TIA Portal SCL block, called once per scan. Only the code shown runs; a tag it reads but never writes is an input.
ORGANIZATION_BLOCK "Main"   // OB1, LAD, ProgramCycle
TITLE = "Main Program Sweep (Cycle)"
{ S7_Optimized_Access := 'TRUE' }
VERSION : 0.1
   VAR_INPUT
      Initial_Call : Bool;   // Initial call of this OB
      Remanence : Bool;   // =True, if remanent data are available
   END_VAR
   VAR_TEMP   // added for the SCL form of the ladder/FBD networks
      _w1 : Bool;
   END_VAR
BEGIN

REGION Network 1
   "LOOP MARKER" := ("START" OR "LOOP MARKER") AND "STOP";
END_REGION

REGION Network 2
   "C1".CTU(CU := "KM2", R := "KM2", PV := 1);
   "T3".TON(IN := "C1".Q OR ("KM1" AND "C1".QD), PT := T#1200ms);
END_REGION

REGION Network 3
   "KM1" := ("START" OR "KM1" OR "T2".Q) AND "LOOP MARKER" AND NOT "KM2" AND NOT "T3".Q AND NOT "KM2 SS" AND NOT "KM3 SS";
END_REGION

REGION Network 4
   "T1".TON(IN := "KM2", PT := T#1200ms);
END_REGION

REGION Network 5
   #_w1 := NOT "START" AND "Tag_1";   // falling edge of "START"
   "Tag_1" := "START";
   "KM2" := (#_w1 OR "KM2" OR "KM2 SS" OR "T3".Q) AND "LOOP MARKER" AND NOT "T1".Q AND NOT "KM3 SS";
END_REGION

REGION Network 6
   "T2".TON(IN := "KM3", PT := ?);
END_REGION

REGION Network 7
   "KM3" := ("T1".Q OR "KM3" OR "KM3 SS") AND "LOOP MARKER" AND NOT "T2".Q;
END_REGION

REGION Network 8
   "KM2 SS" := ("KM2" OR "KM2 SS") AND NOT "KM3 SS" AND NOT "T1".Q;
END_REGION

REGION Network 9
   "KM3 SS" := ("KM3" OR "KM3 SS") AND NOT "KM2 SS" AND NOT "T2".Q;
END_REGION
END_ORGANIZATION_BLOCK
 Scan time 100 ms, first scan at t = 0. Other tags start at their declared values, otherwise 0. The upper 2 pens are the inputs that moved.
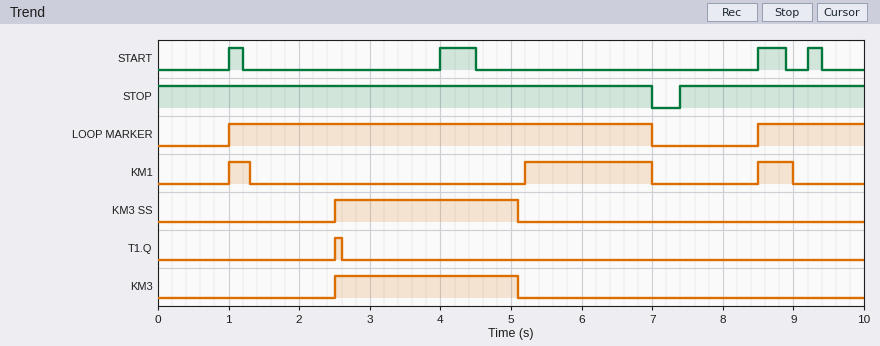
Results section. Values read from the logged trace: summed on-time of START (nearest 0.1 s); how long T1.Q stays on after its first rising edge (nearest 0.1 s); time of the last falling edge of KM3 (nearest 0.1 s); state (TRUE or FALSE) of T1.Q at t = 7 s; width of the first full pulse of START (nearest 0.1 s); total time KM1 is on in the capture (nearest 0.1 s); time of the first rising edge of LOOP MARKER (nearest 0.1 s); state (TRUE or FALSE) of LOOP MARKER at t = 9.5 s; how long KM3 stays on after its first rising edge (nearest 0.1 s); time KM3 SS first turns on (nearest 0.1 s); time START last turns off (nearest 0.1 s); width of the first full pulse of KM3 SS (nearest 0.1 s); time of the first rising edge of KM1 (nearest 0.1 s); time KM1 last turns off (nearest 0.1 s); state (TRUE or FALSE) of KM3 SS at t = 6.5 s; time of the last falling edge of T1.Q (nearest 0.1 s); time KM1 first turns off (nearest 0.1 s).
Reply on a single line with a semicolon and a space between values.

1.3 s; 0.1 s; 5.1 s; FALSE; 0.2 s; 2.6 s; 1.0 s; TRUE; 2.6 s; 2.5 s; 9.4 s; 2.6 s; 1.0 s; 9.0 s; FALSE; 2.6 s; 1.3 s
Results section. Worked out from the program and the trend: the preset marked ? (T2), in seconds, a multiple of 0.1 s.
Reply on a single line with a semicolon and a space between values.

2.5 s
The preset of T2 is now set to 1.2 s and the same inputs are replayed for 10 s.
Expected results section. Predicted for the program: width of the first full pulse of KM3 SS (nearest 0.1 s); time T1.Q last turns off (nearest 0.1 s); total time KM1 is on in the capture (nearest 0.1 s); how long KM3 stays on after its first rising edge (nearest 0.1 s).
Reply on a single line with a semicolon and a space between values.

1.3 s; 5.9 s; 1.1 s; 1.3 s
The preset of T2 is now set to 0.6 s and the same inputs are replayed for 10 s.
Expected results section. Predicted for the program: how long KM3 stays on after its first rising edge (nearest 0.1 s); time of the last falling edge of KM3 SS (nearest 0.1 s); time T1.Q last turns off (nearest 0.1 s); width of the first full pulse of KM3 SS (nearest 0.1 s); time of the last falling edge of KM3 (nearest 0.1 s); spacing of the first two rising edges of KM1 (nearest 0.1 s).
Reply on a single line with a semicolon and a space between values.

0.7 s; 6.5 s; 5.9 s; 0.7 s; 6.5 s; 2.3 s
